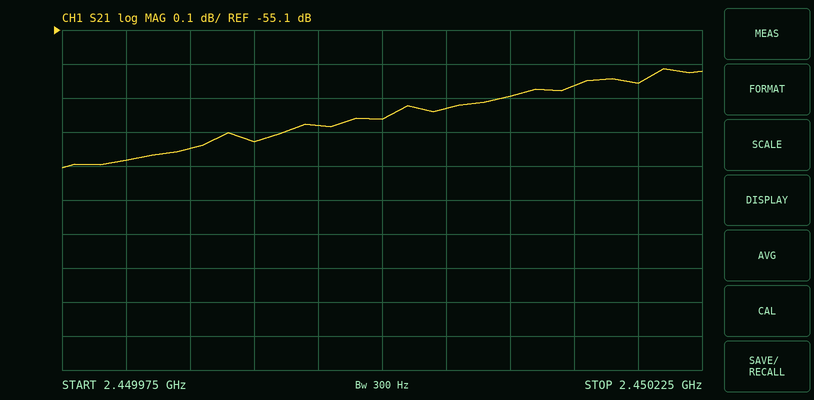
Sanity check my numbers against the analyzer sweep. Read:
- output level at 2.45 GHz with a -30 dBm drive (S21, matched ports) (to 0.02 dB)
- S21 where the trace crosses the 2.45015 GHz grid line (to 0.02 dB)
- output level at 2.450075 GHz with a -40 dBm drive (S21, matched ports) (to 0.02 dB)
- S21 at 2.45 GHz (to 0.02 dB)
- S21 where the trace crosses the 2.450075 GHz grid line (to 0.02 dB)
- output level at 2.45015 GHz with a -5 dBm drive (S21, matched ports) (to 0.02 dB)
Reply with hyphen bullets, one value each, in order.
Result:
- -85.48 dBm
- -55.30 dB
- -95.38 dBm
- -55.48 dB
- -55.38 dB
- -60.30 dBm
